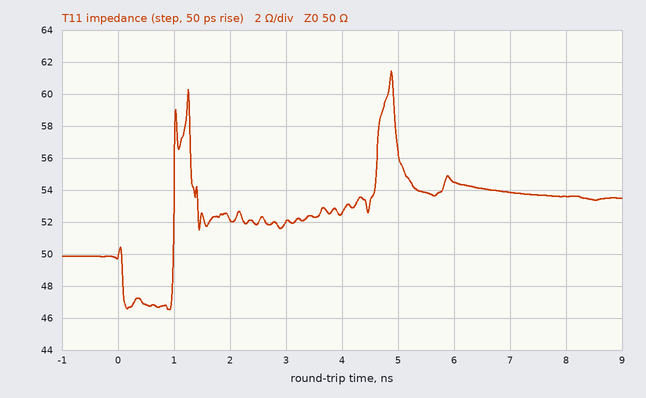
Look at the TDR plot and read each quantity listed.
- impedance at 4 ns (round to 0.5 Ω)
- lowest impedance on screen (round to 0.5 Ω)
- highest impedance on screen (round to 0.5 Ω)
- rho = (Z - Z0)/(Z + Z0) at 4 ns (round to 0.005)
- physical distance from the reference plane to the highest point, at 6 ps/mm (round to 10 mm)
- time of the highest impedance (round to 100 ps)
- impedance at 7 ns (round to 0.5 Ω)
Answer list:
52.5 Ω
46.5 Ω
61.5 Ω
+0.025
410 mm
4.9 ns
54.0 Ω
